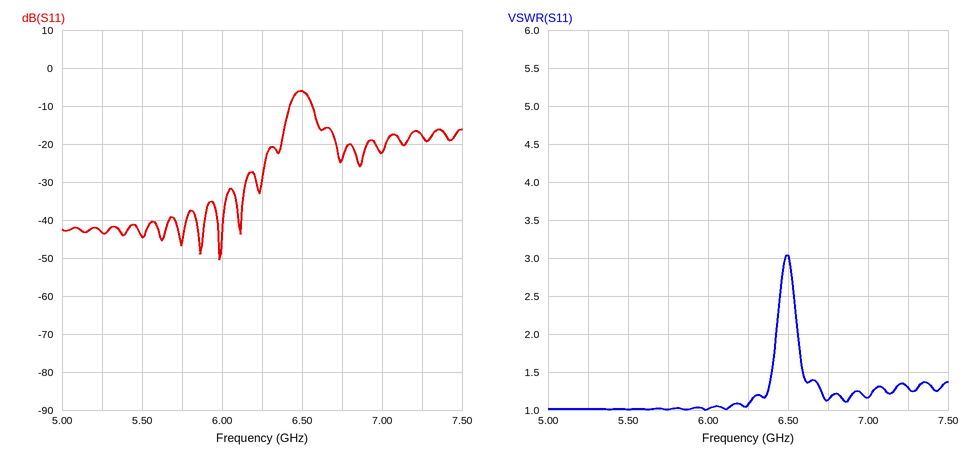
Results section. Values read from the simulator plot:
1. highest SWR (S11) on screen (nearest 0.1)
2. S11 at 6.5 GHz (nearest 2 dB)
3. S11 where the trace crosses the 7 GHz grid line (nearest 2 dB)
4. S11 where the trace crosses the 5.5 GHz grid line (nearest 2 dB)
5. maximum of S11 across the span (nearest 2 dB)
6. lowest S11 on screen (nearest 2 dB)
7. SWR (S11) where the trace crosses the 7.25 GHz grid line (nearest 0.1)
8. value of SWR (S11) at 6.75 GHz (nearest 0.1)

3.0
-6 dB
-22 dB
-44 dB
-6 dB
-50 dB
1.3
1.1
